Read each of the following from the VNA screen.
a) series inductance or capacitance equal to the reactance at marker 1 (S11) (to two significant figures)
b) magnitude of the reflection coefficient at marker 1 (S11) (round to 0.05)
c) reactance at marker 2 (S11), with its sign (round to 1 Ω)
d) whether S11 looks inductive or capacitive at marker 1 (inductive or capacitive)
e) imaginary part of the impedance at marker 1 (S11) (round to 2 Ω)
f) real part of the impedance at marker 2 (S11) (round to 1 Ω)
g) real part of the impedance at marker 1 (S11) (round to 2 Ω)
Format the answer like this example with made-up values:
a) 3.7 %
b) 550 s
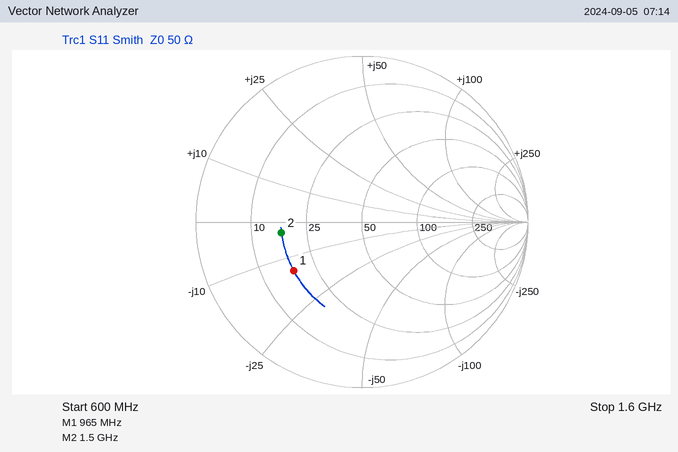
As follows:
a) 12 pF
b) 0.50
c) -3 Ω
d) capacitive
e) -14 Ω
f) 17 Ω
g) 18 Ω
